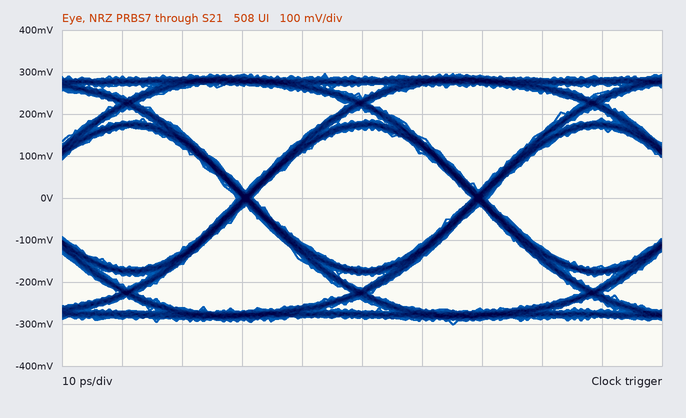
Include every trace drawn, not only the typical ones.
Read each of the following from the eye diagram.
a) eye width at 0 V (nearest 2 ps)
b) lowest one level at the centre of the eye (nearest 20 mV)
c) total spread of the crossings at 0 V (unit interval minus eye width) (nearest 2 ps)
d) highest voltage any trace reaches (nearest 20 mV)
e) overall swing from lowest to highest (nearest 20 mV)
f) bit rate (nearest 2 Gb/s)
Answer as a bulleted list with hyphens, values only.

- 36 ps
- 160 mV
- 2 ps
- 300 mV
- 600 mV
- 26 Gb/s
